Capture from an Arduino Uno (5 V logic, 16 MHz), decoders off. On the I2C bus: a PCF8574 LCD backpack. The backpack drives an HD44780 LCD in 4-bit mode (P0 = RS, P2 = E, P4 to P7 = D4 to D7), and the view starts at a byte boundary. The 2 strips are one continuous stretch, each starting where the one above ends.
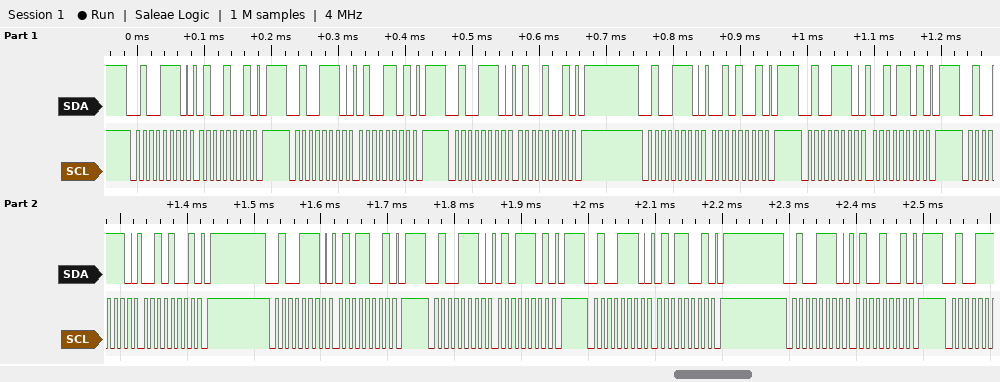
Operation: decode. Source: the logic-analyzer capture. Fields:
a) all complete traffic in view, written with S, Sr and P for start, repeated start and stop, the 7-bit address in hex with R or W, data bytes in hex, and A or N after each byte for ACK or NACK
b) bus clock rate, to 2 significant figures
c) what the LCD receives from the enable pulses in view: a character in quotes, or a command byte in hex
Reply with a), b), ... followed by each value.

a) S 27W A 49 A P S 27W A 4D A P S 27W A 49 A P S 27W A 29 A P S 27W A 2D A P S 27W A 29 A P S 27W A 59 A P S 27W A 5D A P S 27W A 59 A P S 27W A 49 A P
b) 100 kHz
c) 'B'
